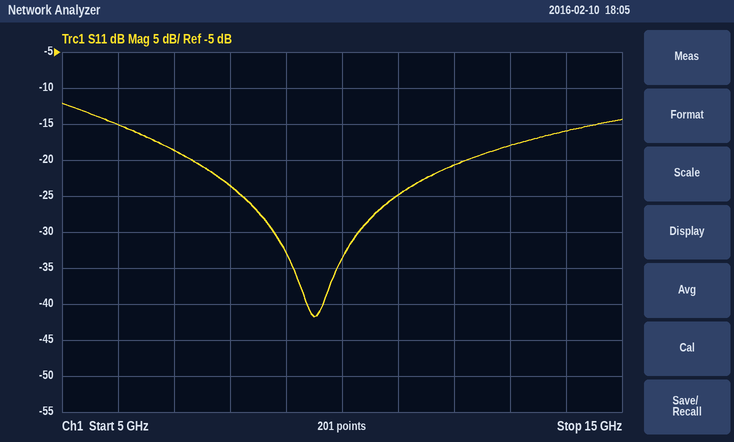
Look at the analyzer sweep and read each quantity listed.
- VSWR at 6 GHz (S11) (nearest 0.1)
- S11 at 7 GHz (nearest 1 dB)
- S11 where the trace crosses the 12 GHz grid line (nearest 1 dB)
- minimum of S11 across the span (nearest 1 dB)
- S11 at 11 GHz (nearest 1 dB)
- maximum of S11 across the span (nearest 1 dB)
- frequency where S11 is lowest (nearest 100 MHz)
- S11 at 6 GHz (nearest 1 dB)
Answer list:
1.4
-19 dB
-21 dB
-42 dB
-25 dB
-12 dB
9.5 GHz
-15 dB
